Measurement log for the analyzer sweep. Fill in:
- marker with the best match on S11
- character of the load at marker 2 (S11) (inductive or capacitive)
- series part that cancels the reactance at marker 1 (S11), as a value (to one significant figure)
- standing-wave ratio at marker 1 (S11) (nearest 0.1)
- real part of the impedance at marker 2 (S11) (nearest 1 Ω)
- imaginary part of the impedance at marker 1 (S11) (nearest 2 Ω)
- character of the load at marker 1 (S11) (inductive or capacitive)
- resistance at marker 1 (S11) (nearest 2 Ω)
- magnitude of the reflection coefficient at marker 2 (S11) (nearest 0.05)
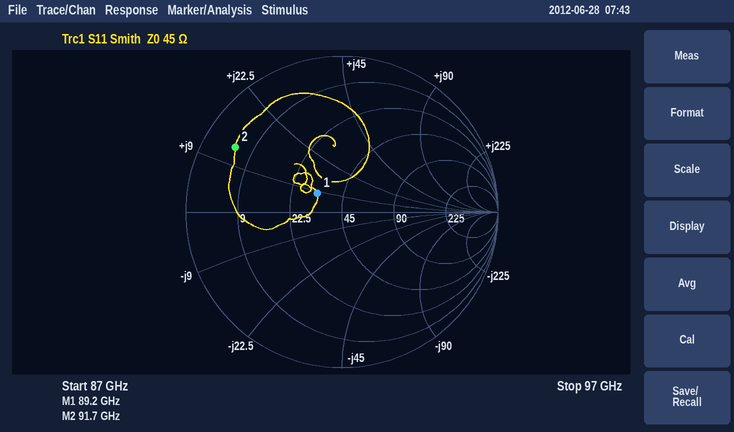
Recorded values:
marker 1
inductive
200 fF
1.5
5 Ω
+8 Ω
inductive
32 Ω
0.80
